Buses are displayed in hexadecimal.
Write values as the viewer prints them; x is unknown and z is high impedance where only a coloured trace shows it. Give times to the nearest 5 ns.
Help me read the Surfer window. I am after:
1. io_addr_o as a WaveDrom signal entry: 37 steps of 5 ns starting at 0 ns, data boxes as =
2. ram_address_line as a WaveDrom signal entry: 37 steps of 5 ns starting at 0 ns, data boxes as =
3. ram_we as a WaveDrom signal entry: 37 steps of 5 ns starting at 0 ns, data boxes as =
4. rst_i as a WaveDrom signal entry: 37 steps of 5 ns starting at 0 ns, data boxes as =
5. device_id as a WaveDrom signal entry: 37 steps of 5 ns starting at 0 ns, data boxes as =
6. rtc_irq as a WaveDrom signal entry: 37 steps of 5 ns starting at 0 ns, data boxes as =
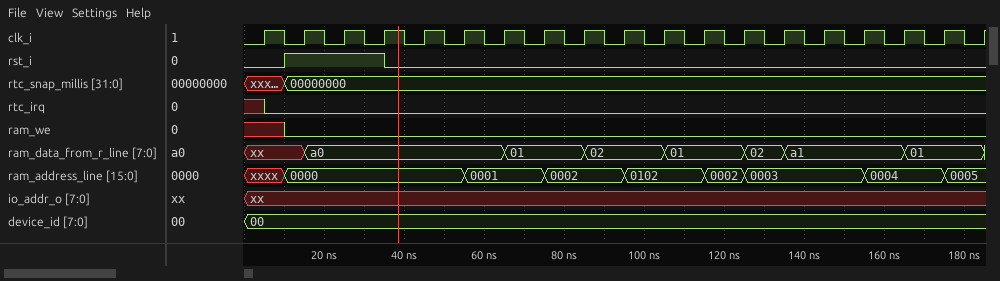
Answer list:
{name: 'io_addr_o', wave: 'x....................................'}
{name: 'ram_address_line', wave: 'x.=........=...=...=...=.=.....=...=.', data: '0000 0001 0002 0102 0002 0003 0004 0005'}
{name: 'ram_we', wave: 'x.0..................................'}
{name: 'rst_i', wave: '0.1....0.............................'}
{name: 'device_id', wave: '=....................................', data: '00'}
{name: 'rtc_irq', wave: 'x0...................................'}
